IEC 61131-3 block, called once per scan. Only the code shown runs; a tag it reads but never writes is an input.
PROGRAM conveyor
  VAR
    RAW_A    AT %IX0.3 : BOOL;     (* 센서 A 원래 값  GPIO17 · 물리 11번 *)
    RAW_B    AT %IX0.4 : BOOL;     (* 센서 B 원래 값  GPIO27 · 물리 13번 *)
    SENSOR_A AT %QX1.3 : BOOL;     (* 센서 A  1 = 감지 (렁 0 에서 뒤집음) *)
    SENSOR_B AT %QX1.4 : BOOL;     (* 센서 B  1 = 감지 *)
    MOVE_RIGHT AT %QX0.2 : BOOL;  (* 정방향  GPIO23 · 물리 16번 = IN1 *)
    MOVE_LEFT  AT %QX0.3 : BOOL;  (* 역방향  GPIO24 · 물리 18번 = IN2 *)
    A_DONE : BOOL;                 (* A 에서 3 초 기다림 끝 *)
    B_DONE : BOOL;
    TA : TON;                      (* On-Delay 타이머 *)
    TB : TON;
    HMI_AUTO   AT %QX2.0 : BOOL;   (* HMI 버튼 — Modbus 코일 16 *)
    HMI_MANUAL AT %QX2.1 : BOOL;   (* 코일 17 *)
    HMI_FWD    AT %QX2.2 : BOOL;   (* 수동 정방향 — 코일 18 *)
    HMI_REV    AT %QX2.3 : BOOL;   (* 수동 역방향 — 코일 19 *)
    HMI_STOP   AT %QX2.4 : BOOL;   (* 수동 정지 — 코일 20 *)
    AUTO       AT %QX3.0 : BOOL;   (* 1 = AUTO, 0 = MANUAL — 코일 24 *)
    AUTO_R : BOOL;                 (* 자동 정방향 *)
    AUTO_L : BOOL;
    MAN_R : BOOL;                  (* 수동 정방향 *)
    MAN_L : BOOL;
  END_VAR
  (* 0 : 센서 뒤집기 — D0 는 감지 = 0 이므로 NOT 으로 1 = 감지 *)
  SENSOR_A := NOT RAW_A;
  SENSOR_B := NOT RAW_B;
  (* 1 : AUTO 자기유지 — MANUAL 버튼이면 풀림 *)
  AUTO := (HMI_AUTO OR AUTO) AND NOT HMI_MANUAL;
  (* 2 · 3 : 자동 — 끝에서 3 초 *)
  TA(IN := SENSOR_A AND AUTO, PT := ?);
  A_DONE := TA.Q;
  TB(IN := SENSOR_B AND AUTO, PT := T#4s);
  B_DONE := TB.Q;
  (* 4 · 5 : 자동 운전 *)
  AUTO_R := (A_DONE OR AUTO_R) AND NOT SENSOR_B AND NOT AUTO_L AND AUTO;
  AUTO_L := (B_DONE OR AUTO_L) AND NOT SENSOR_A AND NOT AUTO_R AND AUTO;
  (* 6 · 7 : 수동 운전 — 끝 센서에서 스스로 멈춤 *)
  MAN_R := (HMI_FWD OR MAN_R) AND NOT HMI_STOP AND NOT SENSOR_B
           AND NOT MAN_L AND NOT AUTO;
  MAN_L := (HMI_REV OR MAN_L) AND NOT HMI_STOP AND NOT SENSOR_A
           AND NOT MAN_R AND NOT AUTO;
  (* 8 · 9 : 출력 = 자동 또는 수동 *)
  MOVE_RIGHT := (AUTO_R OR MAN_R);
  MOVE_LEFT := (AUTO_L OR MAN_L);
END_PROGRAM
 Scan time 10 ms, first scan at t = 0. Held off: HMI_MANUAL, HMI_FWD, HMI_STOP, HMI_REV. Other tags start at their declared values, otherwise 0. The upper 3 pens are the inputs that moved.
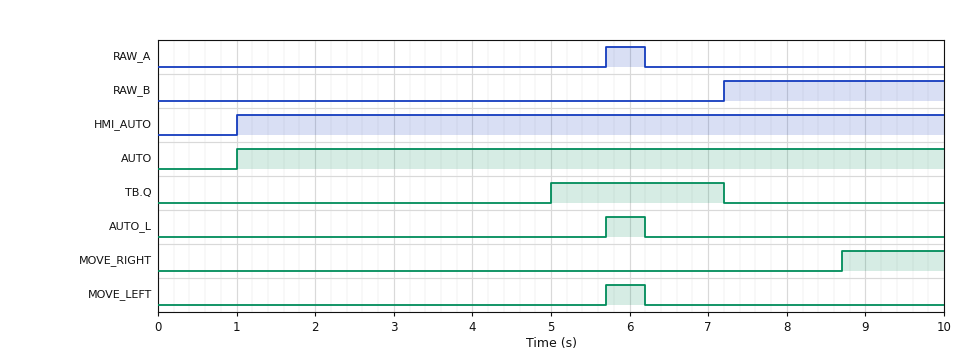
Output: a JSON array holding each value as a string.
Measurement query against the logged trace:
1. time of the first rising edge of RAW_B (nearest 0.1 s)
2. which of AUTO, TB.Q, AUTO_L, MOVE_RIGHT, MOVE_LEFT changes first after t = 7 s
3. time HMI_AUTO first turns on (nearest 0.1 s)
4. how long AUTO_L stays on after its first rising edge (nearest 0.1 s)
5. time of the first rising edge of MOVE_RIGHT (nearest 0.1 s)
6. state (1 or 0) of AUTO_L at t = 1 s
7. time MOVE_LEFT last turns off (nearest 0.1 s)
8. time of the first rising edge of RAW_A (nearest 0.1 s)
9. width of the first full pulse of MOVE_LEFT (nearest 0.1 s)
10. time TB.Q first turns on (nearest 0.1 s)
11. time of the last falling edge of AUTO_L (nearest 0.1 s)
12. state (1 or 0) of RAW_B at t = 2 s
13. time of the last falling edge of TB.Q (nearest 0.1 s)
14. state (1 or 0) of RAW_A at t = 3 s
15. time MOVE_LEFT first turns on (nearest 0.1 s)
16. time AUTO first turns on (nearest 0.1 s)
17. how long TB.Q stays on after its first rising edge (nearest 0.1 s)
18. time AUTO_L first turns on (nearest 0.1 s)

["7.2 s", "TB.Q", "1.0 s", "0.5 s", "8.7 s", "0", "6.2 s", "5.7 s", "0.5 s", "5.0 s", "6.2 s", "0", "7.2 s", "0", "5.7 s", "1.0 s", "2.2 s", "5.7 s"]
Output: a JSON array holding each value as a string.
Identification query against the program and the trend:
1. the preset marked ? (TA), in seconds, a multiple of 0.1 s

["2.5 s"]
